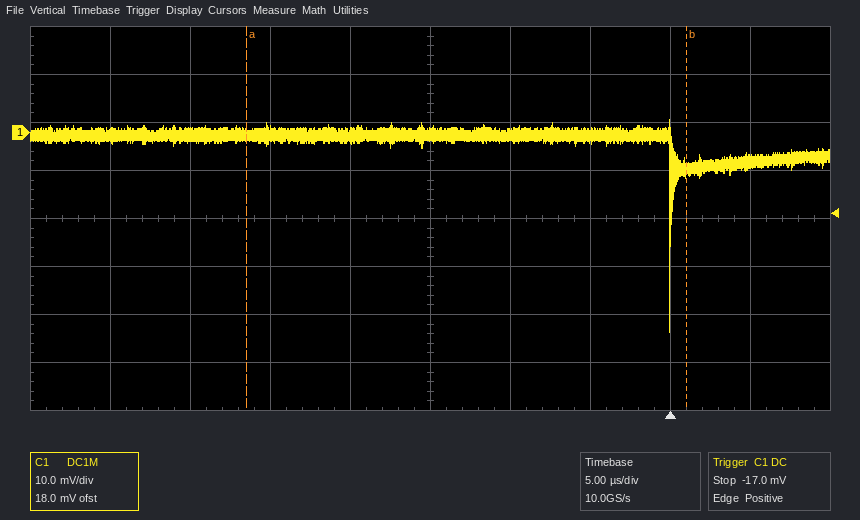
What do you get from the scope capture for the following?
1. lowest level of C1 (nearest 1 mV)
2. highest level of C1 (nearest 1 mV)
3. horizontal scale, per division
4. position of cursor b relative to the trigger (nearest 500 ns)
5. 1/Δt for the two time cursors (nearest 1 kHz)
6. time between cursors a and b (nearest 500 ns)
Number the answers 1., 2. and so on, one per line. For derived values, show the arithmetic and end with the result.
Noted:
1. -42 mV
2. 3 mV
3. 5 µs
4. +1.0 µs
5. 1 / 27.5 µs ≈ 36 kHz
6. 27.5 µs
